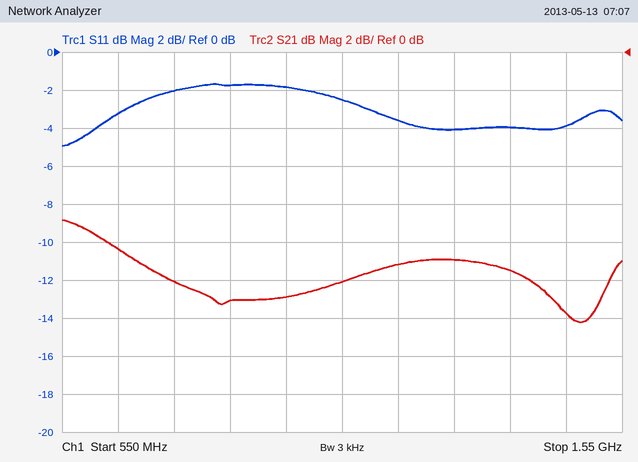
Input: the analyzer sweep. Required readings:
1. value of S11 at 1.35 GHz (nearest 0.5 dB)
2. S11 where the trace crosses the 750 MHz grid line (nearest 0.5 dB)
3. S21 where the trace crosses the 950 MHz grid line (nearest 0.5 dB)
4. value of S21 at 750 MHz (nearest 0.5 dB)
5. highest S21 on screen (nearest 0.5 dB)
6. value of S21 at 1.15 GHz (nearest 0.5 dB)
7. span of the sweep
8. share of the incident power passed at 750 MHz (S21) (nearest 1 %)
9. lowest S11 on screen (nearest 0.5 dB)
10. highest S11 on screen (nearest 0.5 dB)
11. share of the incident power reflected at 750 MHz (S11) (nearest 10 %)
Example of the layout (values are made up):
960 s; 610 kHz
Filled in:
-4.0 dB; -2.0 dB; -13.0 dB; -12.0 dB; -9.0 dB; -11.0 dB; 1 GHz; 6 %; -5.0 dB; -1.5 dB; 60 %
